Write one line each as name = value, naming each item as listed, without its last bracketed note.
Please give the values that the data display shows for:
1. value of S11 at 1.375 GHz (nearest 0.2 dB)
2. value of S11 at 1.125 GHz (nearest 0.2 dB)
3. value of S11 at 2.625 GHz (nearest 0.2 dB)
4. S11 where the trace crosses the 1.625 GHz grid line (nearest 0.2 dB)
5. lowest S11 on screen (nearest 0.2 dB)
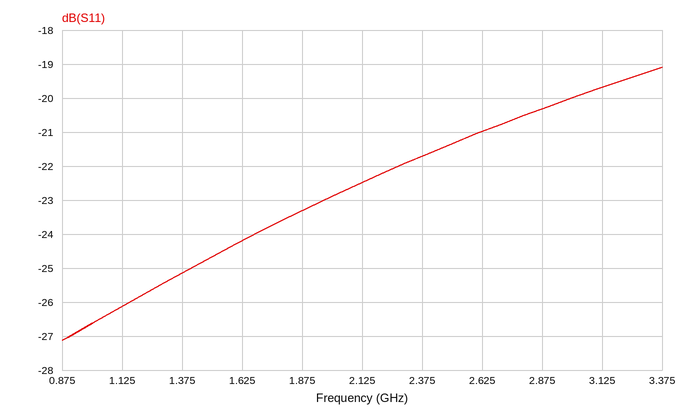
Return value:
value of S11 at 1.375 GHz = -25.2 dB
value of S11 at 1.125 GHz = -26.2 dB
value of S11 at 2.625 GHz = -21.0 dB
S11 where the trace crosses the 1.625 GHz grid line = -24.2 dB
lowest S11 on screen = -27.2 dB
